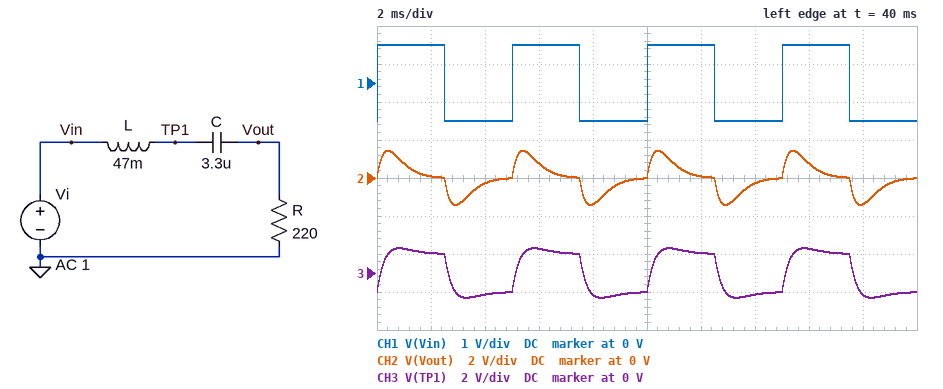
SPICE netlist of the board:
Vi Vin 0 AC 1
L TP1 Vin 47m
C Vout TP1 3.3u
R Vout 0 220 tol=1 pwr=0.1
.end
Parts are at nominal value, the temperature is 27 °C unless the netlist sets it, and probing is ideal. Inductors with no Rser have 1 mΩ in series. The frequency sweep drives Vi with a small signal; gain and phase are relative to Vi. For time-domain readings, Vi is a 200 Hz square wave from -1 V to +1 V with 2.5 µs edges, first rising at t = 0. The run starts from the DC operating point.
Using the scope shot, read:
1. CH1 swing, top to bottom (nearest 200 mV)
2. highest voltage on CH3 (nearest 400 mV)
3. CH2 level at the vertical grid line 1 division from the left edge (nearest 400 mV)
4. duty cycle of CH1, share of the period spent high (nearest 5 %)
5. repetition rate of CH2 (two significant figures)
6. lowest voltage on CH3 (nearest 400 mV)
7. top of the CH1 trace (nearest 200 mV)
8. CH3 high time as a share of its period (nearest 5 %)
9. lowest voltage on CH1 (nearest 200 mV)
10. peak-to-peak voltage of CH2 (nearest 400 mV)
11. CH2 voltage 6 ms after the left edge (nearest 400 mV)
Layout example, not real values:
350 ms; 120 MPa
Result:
2.0 V; 1.2 V; 0 V; 50 %; 200 Hz; -1.2 V; 1.0 V; 50 %; -1.0 V; 2.8 V; 800 mV
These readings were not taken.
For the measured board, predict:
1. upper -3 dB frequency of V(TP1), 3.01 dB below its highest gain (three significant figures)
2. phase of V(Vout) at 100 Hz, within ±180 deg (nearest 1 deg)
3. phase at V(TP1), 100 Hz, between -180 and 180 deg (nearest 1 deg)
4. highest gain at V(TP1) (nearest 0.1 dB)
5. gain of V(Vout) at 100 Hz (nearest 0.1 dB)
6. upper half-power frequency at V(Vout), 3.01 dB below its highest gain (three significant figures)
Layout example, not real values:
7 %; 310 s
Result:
770 Hz; 64 deg; -1 deg; 1.4 dB; -7.2 dB; 922 Hz
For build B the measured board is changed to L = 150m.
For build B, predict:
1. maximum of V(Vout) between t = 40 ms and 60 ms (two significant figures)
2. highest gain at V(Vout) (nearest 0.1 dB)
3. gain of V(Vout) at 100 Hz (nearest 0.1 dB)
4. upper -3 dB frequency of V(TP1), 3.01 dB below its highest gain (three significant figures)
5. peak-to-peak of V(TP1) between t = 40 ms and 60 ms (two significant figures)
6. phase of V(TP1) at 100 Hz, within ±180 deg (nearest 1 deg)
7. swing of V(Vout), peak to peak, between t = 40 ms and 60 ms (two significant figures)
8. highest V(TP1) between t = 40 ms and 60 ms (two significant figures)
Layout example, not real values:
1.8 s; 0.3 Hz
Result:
1.3 V; 0 dB; -6.1 dB; 314 Hz; 3.4 V; -5 deg; 2.6 V; 1.7 V
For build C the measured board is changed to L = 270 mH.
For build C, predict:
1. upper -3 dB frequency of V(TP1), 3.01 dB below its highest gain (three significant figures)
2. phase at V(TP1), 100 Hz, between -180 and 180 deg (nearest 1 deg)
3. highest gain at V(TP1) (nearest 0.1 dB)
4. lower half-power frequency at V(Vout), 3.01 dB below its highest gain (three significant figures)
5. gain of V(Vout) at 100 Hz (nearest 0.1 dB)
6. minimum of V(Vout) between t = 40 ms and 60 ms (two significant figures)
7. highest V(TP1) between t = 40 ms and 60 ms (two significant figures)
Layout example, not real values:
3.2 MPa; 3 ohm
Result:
216 Hz; -11 deg; 4.6 dB; 116 Hz; -4.8 dB; -1.1 V; 1.8 V
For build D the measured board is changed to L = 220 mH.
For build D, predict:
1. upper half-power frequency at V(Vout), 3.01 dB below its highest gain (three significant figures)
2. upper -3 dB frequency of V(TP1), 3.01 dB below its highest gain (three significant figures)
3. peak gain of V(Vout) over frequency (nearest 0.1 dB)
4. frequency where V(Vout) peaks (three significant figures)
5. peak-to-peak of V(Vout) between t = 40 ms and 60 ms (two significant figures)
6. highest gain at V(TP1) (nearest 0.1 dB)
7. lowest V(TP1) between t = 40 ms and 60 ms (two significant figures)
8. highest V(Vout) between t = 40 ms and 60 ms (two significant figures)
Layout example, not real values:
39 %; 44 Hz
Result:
283 Hz; 245 Hz; 0 dB; 187 Hz; 2.4 V; 4.1 dB; -1.8 V; 1.2 V
